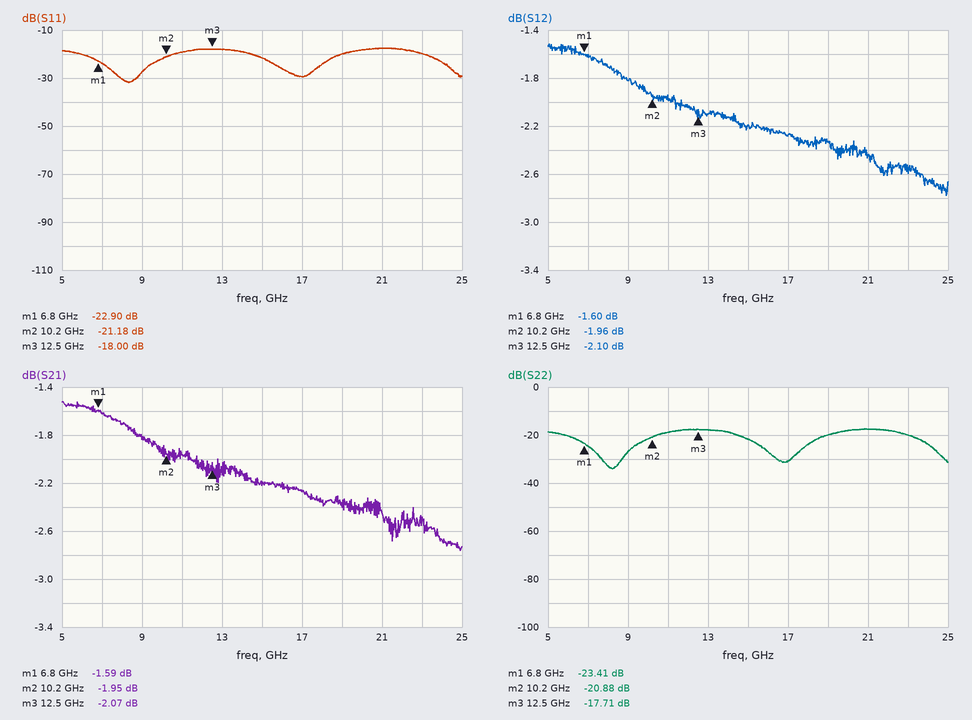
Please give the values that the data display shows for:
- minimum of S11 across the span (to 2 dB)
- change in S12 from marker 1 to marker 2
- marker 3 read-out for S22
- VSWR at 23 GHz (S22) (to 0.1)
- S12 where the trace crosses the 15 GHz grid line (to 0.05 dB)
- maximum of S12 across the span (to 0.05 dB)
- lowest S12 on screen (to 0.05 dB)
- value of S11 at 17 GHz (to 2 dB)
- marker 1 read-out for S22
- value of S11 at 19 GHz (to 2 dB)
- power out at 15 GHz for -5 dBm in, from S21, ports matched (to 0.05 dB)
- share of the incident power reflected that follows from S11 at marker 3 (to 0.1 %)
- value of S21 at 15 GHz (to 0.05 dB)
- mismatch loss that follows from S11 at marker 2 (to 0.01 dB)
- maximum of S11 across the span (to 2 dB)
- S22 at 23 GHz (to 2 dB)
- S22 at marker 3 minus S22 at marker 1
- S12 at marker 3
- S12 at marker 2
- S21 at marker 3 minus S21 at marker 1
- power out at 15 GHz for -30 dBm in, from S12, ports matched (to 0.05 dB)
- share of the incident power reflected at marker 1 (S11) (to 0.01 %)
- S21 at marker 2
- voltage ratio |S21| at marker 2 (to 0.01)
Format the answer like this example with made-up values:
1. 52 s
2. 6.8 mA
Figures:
1. -32 dB
2. -0.36 dB
3. -17.71 dB
4. 1.2
5. -2.20 dB
6. -1.50 dB
7. -2.80 dB
8. -30 dB
9. -23.41 dB
10. -20 dB
11. -7.20 dBm
12. 1.6 %
13. -2.20 dB
14. 0.03 dB
15. -18 dB
16. -20 dB
17. 5.70 dB
18. -2.10 dB
19. -1.96 dB
20. -0.48 dB
21. -32.20 dBm
22. 0.51 %
23. -1.95 dB
24. 0.80
